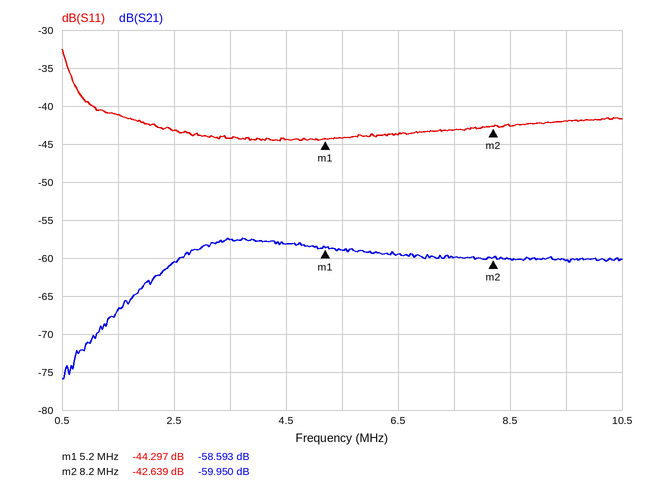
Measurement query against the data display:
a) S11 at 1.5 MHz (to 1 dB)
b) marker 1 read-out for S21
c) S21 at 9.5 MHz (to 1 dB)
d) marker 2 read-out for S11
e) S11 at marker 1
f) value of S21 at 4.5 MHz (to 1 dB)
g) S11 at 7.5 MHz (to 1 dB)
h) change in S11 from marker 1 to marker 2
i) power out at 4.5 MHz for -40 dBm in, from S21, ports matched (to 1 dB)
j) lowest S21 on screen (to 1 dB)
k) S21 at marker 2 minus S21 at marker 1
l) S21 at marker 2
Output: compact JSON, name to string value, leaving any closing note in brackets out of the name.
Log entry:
{"S11 at 1.5 MHz": "-41 dB", "marker 1 read-out for S21": "-58.593 dB", "S21 at 9.5 MHz": "-60 dB", "marker 2 read-out for S11": "-42.639 dB", "S11 at marker 1": "-44.297 dB", "value of S21 at 4.5 MHz": "-58 dB", "S11 at 7.5 MHz": "-43 dB", "change in S11 from marker 1 to marker 2": "1.658 dB", "power out at 4.5 MHz for -40 dBm in, from S21, ports matched": "-98 dBm", "lowest S21 on screen": "-76 dB", "S21 at marker 2 minus S21 at marker 1": "-1.357 dB", "S21 at marker 2": "-59.950 dB"}
